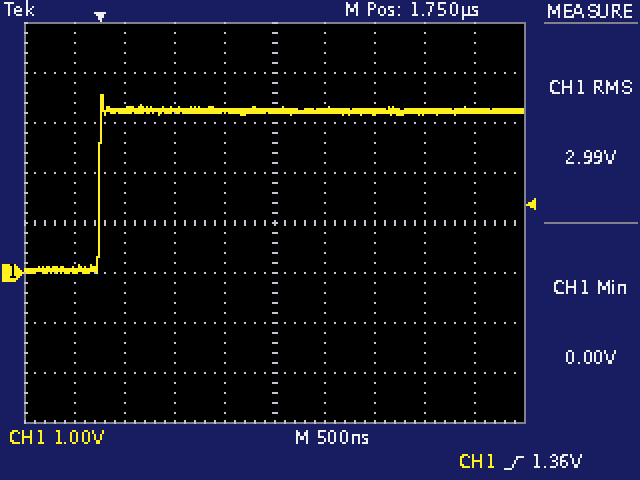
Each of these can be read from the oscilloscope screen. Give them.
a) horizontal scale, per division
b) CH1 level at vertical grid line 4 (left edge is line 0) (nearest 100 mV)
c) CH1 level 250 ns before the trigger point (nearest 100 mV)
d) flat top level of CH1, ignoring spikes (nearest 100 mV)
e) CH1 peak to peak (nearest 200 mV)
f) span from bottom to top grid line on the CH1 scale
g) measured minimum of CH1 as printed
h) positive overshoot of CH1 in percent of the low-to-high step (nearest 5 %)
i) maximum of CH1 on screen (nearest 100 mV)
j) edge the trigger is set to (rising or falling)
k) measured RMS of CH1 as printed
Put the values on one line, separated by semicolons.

500 ns; 3.2 V; 100 mV; 3.2 V; 3.6 V; 8 V; 0.00 V; 10 %; 3.6 V; rising; 2.99 V
